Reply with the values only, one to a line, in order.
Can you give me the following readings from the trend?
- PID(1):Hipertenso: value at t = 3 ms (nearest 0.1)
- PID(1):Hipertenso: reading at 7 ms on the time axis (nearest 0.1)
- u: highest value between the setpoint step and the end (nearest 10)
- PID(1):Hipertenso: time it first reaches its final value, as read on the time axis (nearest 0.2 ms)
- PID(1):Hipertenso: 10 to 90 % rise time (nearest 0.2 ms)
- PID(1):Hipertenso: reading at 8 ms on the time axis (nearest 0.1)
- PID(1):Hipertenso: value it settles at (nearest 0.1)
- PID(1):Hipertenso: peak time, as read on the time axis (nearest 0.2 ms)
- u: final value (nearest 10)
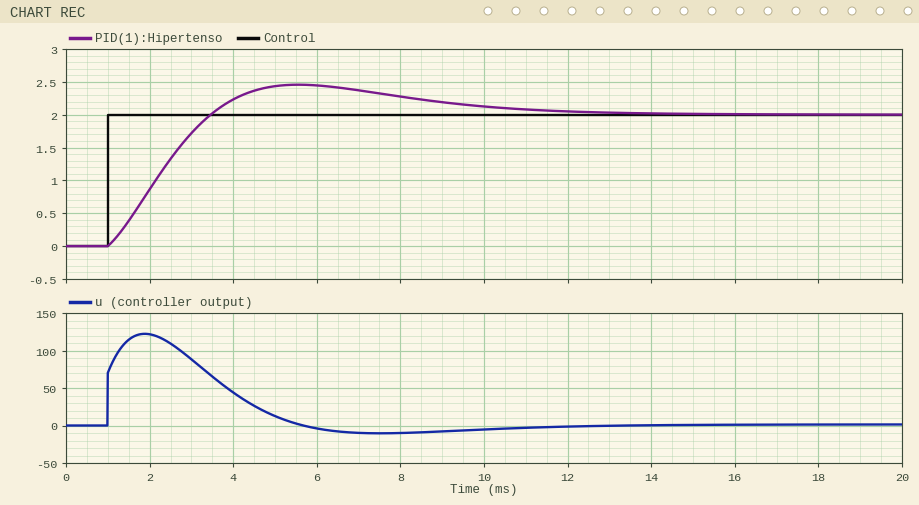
1.7
2.4
120
3.4 ms
1.8 ms
2.3
2.0
5.6 ms
0
